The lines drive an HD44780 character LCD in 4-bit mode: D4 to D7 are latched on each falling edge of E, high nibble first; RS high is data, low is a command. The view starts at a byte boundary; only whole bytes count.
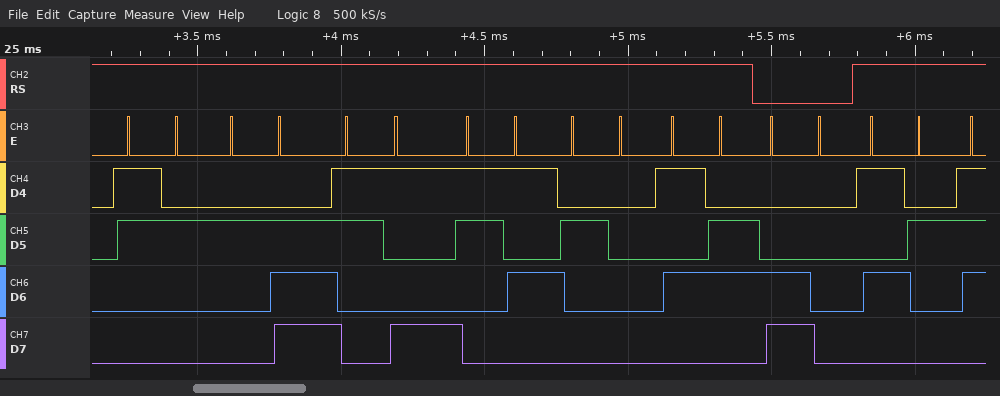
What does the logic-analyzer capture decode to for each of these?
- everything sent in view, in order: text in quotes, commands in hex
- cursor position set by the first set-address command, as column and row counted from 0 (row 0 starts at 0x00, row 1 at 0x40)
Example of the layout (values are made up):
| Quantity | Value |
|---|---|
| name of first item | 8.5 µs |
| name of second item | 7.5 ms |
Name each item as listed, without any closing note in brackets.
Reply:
| Quantity | Value |
|---|---|
| everything sent in view, in order: text in quotes, commands in hex | "2.95 V" 0xC0 "R" |
| cursor position set by the first set-address command, as column and row counted from 0 | column 0, row 1 |
